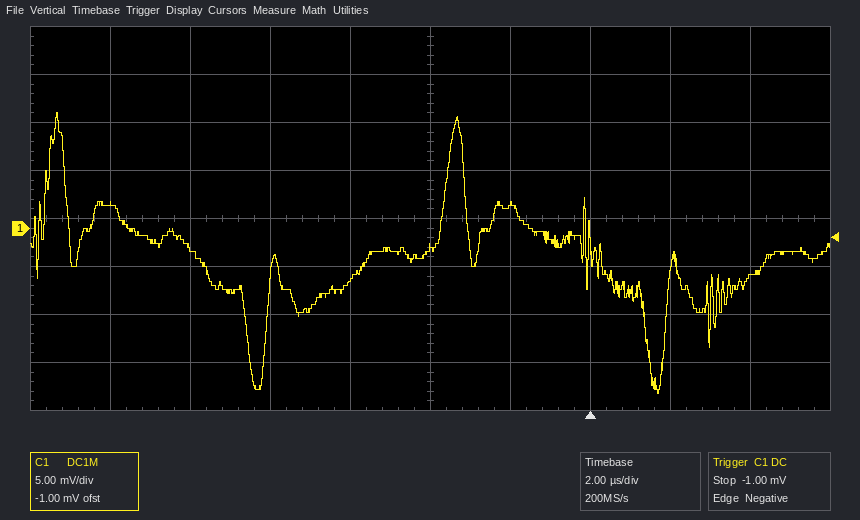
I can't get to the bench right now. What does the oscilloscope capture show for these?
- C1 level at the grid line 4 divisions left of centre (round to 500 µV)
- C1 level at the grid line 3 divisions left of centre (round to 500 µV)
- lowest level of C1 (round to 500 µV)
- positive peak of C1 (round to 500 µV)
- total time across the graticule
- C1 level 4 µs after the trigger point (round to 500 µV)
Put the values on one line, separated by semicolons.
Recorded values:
2.5 mV; -2.0 mV; -17.0 mV; 12.0 mV; 20 µs; -5.0 mV
